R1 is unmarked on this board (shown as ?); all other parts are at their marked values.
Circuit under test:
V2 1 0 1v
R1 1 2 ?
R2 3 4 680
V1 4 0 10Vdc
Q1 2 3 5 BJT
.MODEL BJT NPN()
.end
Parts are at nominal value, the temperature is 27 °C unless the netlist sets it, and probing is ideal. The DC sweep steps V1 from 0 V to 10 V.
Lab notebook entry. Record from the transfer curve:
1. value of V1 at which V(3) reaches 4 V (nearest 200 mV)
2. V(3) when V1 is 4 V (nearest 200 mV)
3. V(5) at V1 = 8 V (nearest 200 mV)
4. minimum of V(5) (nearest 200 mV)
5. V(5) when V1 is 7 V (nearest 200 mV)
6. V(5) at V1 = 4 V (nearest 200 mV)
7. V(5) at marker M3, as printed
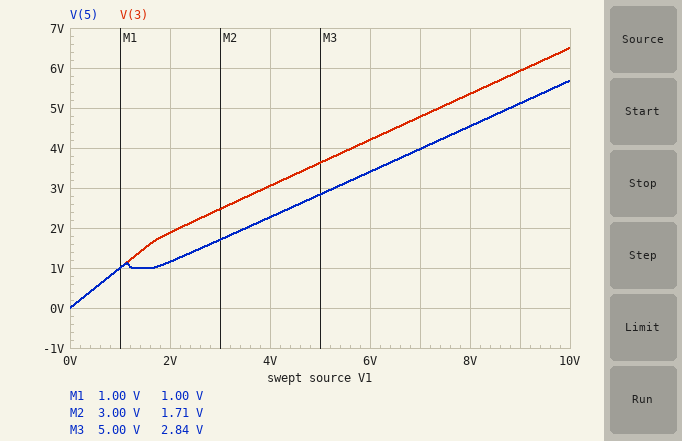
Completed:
5.6 V
3.0 V
4.6 V
0 V
4.0 V
2.2 V
2.84 V
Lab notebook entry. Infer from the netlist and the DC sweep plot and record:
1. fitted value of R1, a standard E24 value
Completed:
910 Ω
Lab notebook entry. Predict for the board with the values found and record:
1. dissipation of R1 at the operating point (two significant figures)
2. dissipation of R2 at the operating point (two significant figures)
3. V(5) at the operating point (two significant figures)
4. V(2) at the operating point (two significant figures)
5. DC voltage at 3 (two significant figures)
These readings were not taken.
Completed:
24 mW
18 mW
5.7 V
5.7 V
6.5 V
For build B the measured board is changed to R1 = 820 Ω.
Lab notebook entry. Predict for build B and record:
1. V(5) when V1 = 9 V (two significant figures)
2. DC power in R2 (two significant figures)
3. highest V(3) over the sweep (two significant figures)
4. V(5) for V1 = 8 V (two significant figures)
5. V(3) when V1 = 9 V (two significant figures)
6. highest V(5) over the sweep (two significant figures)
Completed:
4.9 V
20 mW
6.3 V
4.4 V
5.7 V
5.5 V
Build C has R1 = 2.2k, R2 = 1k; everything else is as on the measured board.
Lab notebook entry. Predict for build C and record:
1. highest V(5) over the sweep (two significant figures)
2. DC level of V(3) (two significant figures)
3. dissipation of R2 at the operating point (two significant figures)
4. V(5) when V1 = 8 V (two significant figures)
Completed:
6.6 V
7.4 V
6.6 mW
5.3 V
